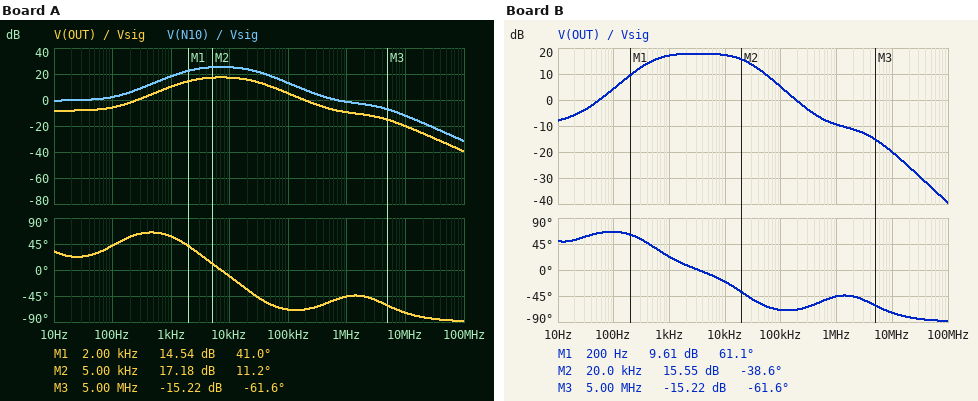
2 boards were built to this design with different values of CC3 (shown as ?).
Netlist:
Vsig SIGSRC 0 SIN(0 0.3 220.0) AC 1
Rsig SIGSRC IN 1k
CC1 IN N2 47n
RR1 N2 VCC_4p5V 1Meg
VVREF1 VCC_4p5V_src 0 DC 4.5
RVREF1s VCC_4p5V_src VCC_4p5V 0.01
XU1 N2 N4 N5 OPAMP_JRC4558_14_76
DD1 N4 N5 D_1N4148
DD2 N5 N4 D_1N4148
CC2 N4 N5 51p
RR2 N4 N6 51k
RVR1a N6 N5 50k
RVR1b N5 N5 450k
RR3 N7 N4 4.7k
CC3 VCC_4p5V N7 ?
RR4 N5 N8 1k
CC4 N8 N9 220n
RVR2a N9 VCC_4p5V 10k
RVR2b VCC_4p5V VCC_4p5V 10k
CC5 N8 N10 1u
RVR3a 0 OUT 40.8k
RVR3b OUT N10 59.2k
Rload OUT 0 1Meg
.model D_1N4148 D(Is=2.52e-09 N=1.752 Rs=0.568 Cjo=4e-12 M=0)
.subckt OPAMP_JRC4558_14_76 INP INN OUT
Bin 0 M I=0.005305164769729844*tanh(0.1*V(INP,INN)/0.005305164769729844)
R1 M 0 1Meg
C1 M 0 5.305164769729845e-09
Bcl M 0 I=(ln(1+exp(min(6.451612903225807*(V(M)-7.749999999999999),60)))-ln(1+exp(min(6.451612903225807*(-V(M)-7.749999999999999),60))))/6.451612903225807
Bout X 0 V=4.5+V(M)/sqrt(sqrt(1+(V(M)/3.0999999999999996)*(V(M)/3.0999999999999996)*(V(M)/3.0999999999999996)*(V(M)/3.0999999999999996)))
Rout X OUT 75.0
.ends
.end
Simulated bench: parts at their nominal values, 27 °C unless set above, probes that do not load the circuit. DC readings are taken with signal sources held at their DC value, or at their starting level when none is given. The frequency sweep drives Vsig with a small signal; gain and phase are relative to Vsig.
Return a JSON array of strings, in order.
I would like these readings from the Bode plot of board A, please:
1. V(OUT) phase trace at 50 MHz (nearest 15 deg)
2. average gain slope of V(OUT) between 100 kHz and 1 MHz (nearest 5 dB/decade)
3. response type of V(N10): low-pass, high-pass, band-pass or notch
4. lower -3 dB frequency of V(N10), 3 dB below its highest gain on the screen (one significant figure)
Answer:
["-90 deg", "-15 dB/decade", "band-pass", "2 kHz"]
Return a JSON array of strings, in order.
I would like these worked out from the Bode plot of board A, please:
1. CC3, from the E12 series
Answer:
["15 nF"]
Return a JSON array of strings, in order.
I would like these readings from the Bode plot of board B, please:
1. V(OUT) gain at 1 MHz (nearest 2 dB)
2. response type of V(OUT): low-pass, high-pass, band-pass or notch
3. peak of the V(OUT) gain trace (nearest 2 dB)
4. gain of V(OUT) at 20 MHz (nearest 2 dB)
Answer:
["-10 dB", "band-pass", "18 dB", "-26 dB"]
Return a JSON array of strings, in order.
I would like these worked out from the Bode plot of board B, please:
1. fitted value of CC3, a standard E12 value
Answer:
["68 nF"]
